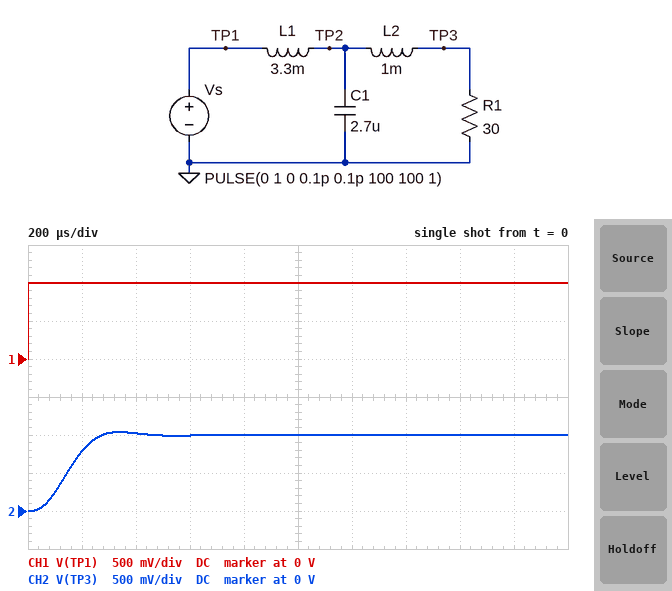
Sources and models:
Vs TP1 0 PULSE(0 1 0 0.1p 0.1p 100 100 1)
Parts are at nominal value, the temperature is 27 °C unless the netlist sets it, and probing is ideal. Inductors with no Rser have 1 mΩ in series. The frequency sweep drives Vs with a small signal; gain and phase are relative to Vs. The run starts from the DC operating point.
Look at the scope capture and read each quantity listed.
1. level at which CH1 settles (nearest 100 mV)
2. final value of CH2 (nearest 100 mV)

1.0 V
1.0 V
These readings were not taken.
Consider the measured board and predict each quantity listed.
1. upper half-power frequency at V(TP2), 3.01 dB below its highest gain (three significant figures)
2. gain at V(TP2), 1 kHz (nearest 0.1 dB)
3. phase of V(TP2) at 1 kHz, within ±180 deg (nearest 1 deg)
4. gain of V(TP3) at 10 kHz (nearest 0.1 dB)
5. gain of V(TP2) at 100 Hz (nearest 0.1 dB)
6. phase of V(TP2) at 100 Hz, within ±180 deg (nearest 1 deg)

2.46 kHz
-0.2 dB
-40 deg
-37.3 dB
0 dB
-4 deg
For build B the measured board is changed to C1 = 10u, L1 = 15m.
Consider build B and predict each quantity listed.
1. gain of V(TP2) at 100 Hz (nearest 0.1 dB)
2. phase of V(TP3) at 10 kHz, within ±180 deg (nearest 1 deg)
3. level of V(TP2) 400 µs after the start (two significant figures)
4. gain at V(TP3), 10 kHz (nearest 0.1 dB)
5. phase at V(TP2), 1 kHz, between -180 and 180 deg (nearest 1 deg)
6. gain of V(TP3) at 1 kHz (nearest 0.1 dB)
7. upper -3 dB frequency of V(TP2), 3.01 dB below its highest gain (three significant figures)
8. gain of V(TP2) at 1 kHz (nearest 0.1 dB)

0 dB
116 deg
350 mV
-62.6 dB
-145 deg
-14.6 dB
453 Hz
-14.4 dB
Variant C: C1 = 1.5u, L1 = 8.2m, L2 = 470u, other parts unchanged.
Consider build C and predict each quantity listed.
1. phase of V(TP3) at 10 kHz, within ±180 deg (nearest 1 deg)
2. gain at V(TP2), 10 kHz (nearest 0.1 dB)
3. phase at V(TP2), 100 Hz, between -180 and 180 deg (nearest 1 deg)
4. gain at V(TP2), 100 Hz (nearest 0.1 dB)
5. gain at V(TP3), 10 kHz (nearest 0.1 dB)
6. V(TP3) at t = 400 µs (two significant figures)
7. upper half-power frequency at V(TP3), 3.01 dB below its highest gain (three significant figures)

148 deg
-32.0 dB
-10 deg
-0.1 dB
-35.0 dB
770 mV
652 Hz
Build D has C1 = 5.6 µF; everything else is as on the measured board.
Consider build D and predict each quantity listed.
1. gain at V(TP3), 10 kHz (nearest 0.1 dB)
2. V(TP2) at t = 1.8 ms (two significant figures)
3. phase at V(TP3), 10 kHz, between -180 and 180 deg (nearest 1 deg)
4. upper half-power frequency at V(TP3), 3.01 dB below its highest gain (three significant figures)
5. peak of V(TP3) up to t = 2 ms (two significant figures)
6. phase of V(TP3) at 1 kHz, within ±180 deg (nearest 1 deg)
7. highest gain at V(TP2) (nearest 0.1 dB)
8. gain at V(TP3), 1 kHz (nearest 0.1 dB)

-44.1 dB
1.0 V
117 deg
1.55 kHz
1.2 V
-70 deg
2.2 dB
2.0 dB
